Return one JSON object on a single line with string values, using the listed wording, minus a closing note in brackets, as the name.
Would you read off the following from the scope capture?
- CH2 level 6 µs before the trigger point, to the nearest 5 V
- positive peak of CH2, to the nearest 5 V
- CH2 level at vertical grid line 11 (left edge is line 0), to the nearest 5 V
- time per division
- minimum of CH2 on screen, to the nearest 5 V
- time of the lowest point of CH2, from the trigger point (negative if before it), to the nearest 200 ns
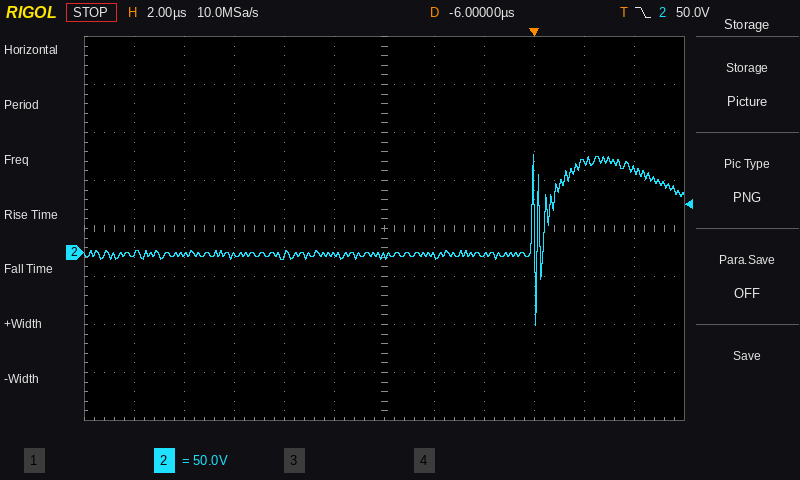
{"CH2 level 6 µs before the trigger point, to the nearest 5 V": "-5 V", "positive peak of CH2, to the nearest 5 V": "100 V", "CH2 level at vertical grid line 11 (left edge is line 0), to the nearest 5 V": "85 V", "time per division": "2 µs", "minimum of CH2 on screen, to the nearest 5 V": "-75 V", "time of the lowest point of CH2, from the trigger point (negative if before it), to the nearest 200 ns": "0.0 µs"}
